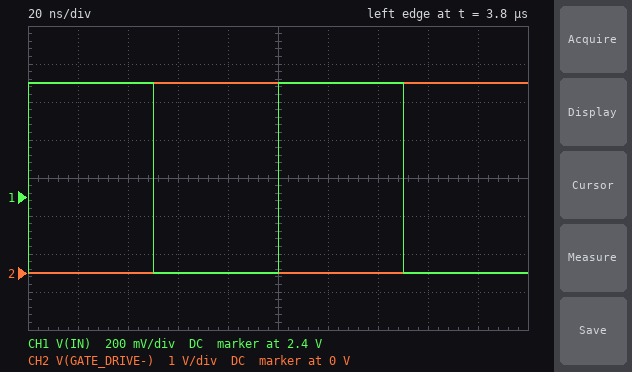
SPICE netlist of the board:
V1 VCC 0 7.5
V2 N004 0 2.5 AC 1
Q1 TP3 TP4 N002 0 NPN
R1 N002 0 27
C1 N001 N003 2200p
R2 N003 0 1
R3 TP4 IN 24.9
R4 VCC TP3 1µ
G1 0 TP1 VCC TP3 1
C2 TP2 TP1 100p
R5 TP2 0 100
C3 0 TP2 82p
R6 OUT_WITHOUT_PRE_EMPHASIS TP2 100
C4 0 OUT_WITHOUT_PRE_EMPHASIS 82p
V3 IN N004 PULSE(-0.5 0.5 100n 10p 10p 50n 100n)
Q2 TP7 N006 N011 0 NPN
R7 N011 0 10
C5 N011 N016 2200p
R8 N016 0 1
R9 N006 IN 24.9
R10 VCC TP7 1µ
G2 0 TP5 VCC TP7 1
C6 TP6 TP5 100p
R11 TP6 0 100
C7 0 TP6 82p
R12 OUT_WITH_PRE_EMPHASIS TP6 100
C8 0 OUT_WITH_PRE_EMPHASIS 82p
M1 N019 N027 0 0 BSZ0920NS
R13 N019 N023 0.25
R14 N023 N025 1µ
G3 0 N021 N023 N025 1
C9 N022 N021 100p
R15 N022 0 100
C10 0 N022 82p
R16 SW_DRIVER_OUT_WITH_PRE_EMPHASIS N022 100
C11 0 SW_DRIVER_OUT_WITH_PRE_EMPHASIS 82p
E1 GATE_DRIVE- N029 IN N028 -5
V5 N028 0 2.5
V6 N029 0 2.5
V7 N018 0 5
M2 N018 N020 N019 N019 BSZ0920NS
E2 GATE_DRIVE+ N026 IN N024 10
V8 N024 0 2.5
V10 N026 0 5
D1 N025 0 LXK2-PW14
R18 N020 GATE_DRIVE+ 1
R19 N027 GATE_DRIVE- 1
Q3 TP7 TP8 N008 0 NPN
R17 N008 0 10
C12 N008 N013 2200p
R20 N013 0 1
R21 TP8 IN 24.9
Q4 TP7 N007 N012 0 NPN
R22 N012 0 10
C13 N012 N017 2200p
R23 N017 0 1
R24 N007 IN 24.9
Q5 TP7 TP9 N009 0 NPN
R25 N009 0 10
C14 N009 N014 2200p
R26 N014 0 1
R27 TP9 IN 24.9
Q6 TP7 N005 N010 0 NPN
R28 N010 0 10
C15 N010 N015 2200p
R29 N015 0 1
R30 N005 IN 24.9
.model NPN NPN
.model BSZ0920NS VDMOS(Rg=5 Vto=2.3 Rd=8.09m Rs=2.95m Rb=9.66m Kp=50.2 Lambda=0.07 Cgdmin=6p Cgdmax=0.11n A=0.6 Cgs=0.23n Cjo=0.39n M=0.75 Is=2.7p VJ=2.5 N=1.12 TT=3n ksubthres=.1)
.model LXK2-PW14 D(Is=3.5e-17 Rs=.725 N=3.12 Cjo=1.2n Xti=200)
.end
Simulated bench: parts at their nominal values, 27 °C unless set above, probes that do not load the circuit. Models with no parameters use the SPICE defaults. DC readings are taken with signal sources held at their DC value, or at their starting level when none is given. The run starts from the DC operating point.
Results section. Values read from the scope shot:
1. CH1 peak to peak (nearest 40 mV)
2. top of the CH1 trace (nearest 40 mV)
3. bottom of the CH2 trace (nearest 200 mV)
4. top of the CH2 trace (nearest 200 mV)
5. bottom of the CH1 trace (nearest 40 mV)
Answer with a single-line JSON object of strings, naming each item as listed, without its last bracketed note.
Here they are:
{"CH1 peak to peak": "1.00 V", "top of the CH1 trace": "3.00 V", "bottom of the CH2 trace": "0 V", "top of the CH2 trace": "5.0 V", "bottom of the CH1 trace": "2.00 V"}
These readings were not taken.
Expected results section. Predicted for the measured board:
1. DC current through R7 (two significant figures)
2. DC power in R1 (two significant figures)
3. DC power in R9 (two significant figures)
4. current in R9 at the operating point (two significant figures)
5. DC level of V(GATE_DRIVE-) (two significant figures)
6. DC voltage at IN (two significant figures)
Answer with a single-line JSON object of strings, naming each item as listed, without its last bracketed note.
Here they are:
{"DC current through R7": "110 mA", "DC power in R1": "46 mW", "DC power in R9": "28 µW", "current in R9 at the operating point": "1.1 mA", "DC level of V(GATE_DRIVE-)": "5.0 V", "DC voltage at IN": "2.0 V"}
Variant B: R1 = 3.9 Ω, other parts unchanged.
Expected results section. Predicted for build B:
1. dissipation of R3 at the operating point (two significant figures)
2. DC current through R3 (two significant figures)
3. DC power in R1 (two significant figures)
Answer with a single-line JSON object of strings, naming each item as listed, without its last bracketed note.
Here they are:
{"dissipation of R3 at the operating point": "170 µW", "DC current through R3": "2.6 mA", "DC power in R1": "270 mW"}
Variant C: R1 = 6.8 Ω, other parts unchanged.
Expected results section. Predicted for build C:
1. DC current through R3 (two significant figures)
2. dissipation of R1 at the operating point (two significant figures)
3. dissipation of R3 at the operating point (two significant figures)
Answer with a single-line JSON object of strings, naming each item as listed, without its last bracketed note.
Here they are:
{"DC current through R3": "1.5 mA", "dissipation of R1 at the operating point": "160 mW", "dissipation of R3 at the operating point": "59 µW"}
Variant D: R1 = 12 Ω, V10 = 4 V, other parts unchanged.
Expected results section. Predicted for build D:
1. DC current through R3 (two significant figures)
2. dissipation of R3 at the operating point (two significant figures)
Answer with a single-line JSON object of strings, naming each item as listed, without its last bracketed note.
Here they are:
{"DC current through R3": "900 µA", "dissipation of R3 at the operating point": "20 µW"}
